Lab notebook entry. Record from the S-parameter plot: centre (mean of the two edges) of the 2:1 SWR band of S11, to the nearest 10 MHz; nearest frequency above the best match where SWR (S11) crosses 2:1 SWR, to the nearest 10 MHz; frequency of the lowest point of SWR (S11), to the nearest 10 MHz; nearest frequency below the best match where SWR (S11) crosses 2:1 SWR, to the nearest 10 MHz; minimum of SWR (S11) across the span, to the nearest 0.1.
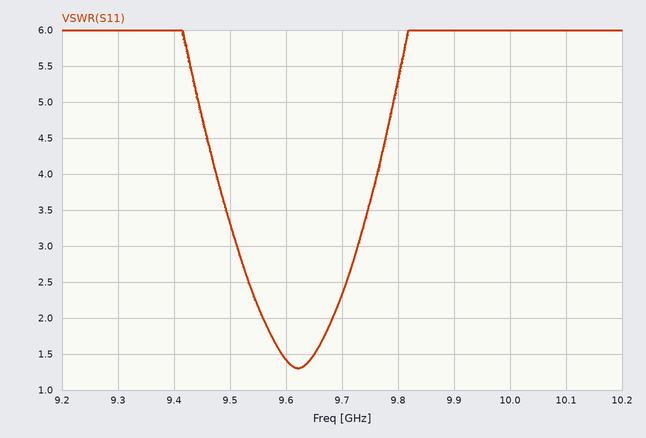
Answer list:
9.62 GHz
9.68 GHz
9.62 GHz
9.56 GHz
1.3
